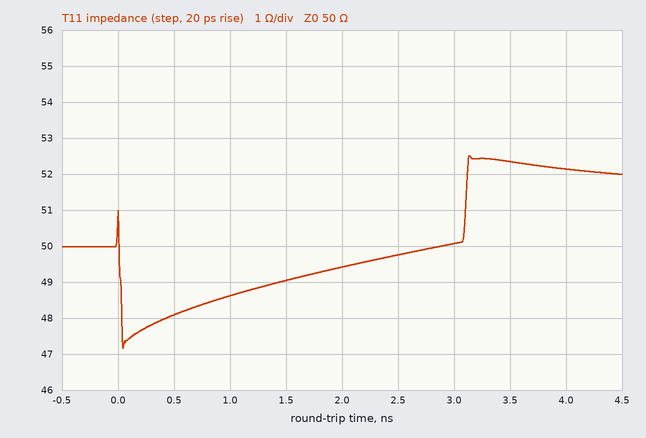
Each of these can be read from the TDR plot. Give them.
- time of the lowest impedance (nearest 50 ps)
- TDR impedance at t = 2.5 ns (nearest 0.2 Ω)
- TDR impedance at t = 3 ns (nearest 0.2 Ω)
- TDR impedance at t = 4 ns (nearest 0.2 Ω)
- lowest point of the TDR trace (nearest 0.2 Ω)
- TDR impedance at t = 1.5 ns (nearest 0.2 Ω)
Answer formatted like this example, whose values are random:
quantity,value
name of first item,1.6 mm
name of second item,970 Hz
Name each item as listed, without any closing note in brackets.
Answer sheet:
quantity,value
time of the lowest impedance,50 ps
TDR impedance at t = 2.5 ns,49.8 Ω
TDR impedance at t = 3 ns,50.0 Ω
TDR impedance at t = 4 ns,52.2 Ω
lowest point of the TDR trace,47.2 Ω
TDR impedance at t = 1.5 ns,49.0 Ω
